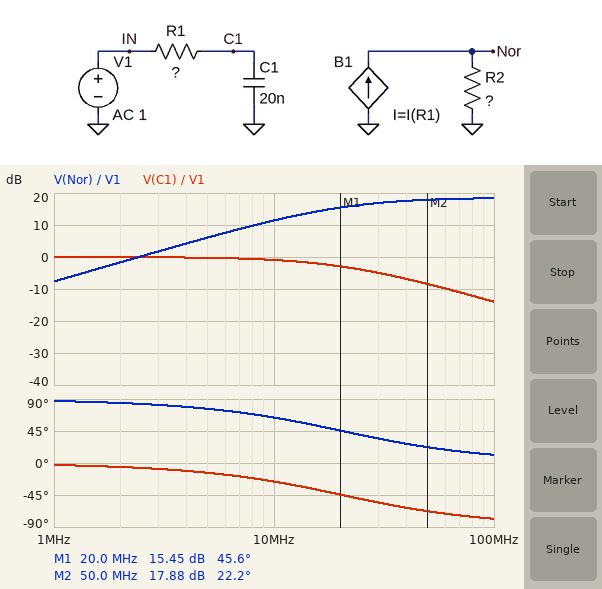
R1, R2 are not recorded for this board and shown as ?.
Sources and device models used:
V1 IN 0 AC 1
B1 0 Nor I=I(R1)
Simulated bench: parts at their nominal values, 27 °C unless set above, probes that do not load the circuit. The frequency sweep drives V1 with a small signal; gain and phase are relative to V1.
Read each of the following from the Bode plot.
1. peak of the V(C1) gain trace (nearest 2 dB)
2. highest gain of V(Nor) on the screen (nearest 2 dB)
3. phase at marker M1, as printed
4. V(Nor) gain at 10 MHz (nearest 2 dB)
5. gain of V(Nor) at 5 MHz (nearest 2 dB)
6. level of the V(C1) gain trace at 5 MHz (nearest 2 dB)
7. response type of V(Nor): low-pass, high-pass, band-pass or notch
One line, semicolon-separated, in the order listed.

0 dB; 18 dB; 45.6 deg; 12 dB; 6 dB; 0 dB; high-pass
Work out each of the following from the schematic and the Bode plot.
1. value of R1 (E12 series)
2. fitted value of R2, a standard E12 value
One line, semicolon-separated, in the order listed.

0.39 Ω; 3.3 Ω
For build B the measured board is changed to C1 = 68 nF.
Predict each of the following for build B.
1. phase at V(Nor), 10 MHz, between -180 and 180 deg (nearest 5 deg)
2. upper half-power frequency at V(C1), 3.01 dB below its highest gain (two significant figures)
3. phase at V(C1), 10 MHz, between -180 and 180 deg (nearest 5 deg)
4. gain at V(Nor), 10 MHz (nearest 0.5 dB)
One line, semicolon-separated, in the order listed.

30 deg; 6.0 MHz; -60 deg; 17.0 dB
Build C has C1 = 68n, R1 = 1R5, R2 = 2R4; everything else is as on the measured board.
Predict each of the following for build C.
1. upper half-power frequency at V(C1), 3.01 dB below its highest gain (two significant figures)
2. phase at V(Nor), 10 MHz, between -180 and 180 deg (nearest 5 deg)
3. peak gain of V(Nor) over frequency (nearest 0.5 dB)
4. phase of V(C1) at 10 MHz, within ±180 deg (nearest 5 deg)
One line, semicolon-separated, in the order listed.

1.6 MHz; 10 deg; 4.0 dB; -80 deg
